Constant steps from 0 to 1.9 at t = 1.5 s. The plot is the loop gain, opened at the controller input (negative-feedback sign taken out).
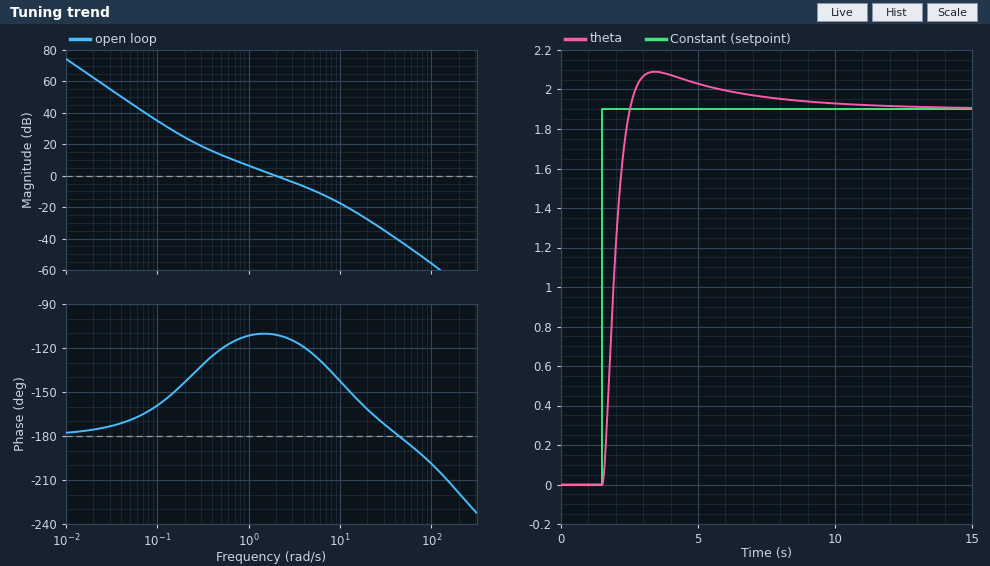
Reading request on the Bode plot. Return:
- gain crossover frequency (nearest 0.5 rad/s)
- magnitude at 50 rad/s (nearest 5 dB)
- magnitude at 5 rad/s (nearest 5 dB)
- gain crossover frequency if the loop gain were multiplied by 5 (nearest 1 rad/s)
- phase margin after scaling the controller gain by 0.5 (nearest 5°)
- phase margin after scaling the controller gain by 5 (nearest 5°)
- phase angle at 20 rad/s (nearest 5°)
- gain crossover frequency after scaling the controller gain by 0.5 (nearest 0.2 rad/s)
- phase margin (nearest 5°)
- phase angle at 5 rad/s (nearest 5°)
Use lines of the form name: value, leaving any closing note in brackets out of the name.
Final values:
gain crossover frequency: 2.0 rad/s
magnitude at 50 rad/s: -45 dB
magnitude at 5 rad/s: -10 dB
gain crossover frequency if the loop gain were multiplied by 5: 8 rad/s
phase margin after scaling the controller gain by 0.5: 70°
phase margin after scaling the controller gain by 5: 45°
phase angle at 20 rad/s: -160°
gain crossover frequency after scaling the controller gain by 0.5: 1.0 rad/s
phase margin: 70°
phase angle at 5 rad/s: -125°
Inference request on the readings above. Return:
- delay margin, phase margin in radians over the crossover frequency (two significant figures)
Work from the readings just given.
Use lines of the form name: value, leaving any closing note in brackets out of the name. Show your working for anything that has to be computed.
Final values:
delay margin, phase margin in radians over the crossover frequency: 70 × π / 180 / 2 = 0.61 s
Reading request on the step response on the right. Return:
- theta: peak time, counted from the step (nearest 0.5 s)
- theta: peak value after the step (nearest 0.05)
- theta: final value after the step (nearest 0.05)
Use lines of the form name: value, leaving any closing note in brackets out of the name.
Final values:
theta: peak time, counted from the step: 2.0 s
theta: peak value after the step: 2.10
theta: final value after the step: 1.90
